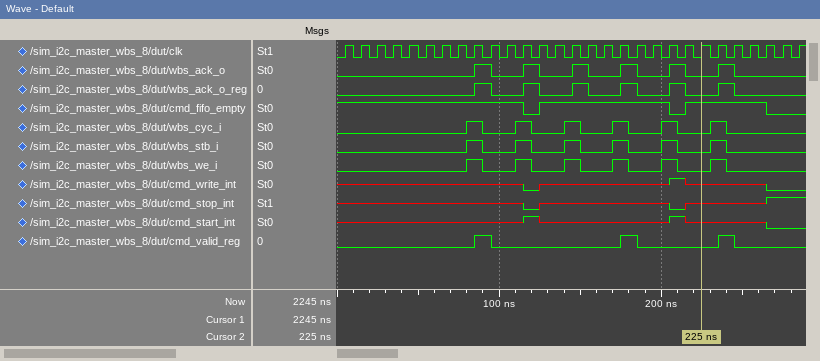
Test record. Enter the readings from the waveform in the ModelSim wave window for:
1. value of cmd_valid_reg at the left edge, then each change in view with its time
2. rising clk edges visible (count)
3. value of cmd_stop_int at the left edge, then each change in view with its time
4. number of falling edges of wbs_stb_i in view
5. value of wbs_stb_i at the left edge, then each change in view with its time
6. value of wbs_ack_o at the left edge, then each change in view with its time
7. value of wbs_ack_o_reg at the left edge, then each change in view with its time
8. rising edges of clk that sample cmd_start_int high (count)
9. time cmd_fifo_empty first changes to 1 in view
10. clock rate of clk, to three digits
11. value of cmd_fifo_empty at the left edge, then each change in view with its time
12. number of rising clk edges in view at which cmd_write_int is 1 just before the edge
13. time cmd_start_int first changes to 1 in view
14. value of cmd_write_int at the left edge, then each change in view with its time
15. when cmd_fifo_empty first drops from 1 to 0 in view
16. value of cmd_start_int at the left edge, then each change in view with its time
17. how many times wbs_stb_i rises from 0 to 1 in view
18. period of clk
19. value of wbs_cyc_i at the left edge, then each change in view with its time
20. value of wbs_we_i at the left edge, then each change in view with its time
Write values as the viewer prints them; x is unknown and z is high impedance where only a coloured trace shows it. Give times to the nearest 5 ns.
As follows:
0, 1 at 85 ns, 0 at 95 ns, 1 at 175 ns, 0 at 185 ns, 1 at 235 ns, 0 at 245 ns
29
x, 0 at 115 ns, x at 125 ns, 0 at 205 ns, x at 215 ns, 1 at 265 ns
6
0, 1 at 80 ns, 0 at 90 ns, 1 at 110 ns, 0 at 120 ns, 1 at 140 ns, 0 at 150 ns, 1 at 170 ns, 0 at 180 ns, 1 at 200 ns, 0 at 210 ns, 1 at 230 ns, 0 at 240 ns
0, 1 at 85 ns, 0 at 95 ns, 1 at 115 ns, 0 at 125 ns, 1 at 145 ns, 0 at 155 ns, 1 at 175 ns, 0 at 185 ns, 1 at 205 ns, 0 at 215 ns, 1 at 235 ns, 0 at 245 ns
0, 1 at 85 ns, 0 at 95 ns, 1 at 115 ns, 0 at 125 ns, 1 at 145 ns, 0 at 155 ns, 1 at 175 ns, 0 at 185 ns, 1 at 205 ns, 0 at 215 ns, 1 at 235 ns, 0 at 245 ns
2
125 ns
100 MHz
1, 0 at 115 ns, 1 at 125 ns, 0 at 205 ns, 1 at 215 ns, 0 at 265 ns
1
115 ns
x, 0 at 115 ns, x at 125 ns, 1 at 205 ns, x at 215 ns, 0 at 265 ns
115 ns
x, 1 at 115 ns, x at 125 ns, 1 at 205 ns, x at 215 ns, 0 at 265 ns
6
10 ns
0, 1 at 80 ns, 0 at 90 ns, 1 at 110 ns, 0 at 120 ns, 1 at 140 ns, 0 at 150 ns, 1 at 170 ns, 0 at 180 ns, 1 at 200 ns, 0 at 210 ns, 1 at 230 ns, 0 at 240 ns
0, 1 at 80 ns, 0 at 90 ns, 1 at 110 ns, 0 at 120 ns, 1 at 140 ns, 0 at 150 ns, 1 at 170 ns, 0 at 180 ns, 1 at 200 ns, 0 at 210 ns, 1 at 230 ns, 0 at 240 ns
